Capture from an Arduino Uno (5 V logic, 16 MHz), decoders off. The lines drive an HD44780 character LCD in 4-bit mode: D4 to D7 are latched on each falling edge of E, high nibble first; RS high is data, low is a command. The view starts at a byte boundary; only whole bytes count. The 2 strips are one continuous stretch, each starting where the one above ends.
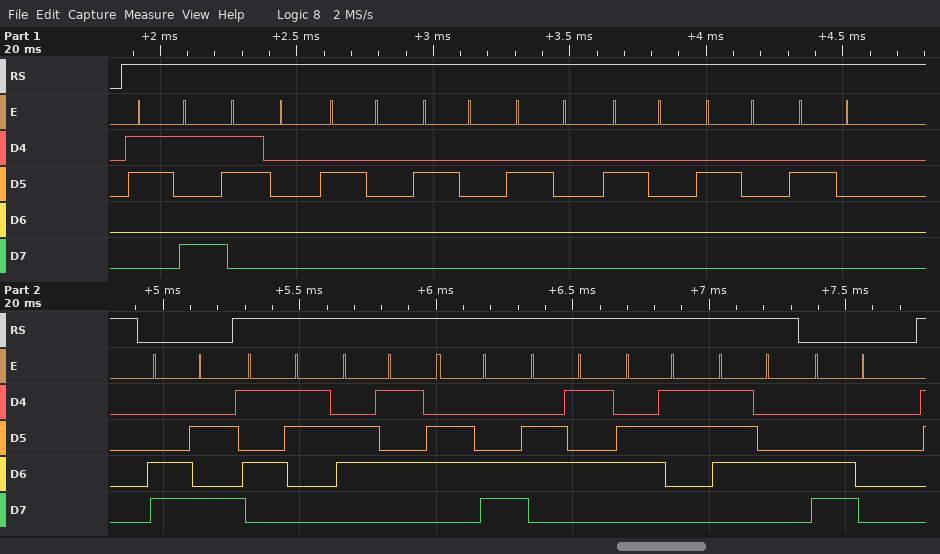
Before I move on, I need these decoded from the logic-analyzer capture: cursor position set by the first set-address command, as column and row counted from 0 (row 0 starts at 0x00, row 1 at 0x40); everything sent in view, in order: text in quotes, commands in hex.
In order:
column 10, row 1
"90      " 0xCA "Select" 0xC0
